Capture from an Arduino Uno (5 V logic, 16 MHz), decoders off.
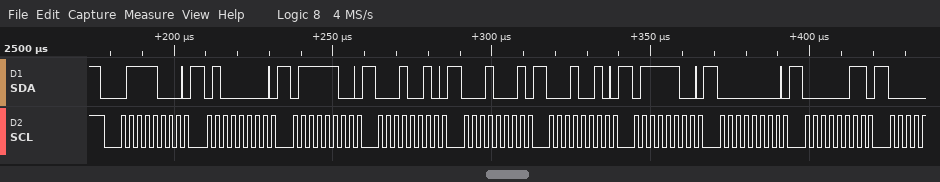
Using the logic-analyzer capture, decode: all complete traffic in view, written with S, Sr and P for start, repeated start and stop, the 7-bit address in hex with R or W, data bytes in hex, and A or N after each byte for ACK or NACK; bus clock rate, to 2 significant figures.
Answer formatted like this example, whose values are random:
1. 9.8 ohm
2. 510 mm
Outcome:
1. S 3CW A 40 A 7C A 12 A 11 A 12 A 7C A 00 A 03 A
2. 400 kHz
